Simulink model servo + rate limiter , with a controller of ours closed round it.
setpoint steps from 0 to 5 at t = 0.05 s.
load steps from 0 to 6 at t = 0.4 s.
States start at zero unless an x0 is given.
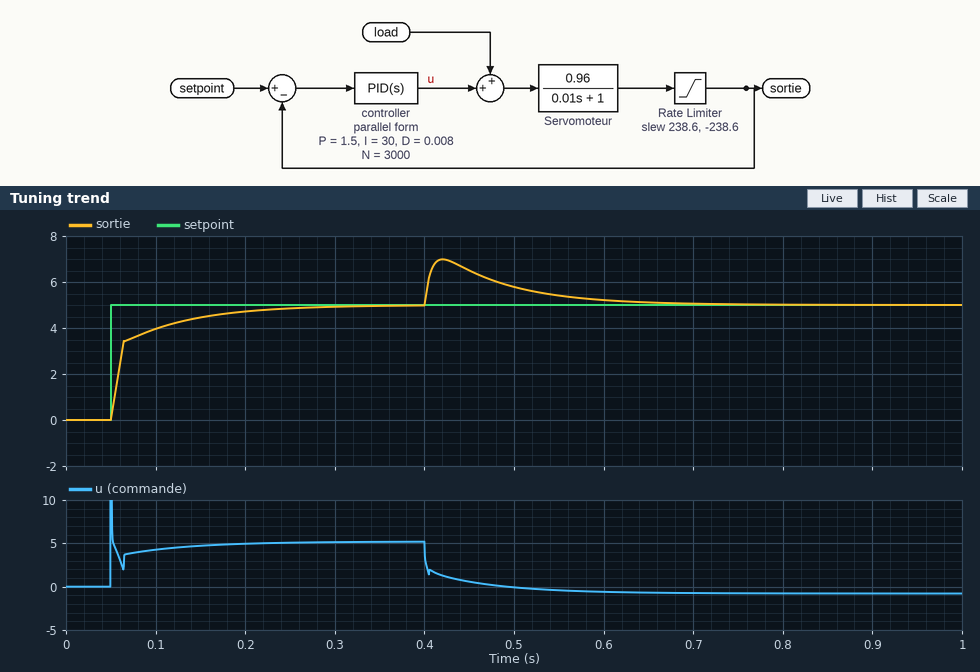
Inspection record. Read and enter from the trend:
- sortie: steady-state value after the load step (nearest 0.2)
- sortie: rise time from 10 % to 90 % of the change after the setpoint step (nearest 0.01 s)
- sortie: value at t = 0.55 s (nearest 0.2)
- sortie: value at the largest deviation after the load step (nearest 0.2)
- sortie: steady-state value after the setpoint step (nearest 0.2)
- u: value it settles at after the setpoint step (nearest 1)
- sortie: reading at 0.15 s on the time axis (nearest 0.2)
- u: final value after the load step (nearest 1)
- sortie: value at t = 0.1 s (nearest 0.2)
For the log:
5.0
0.10 s
5.4
7.0
5.0
5
4.4
-1
4.0
